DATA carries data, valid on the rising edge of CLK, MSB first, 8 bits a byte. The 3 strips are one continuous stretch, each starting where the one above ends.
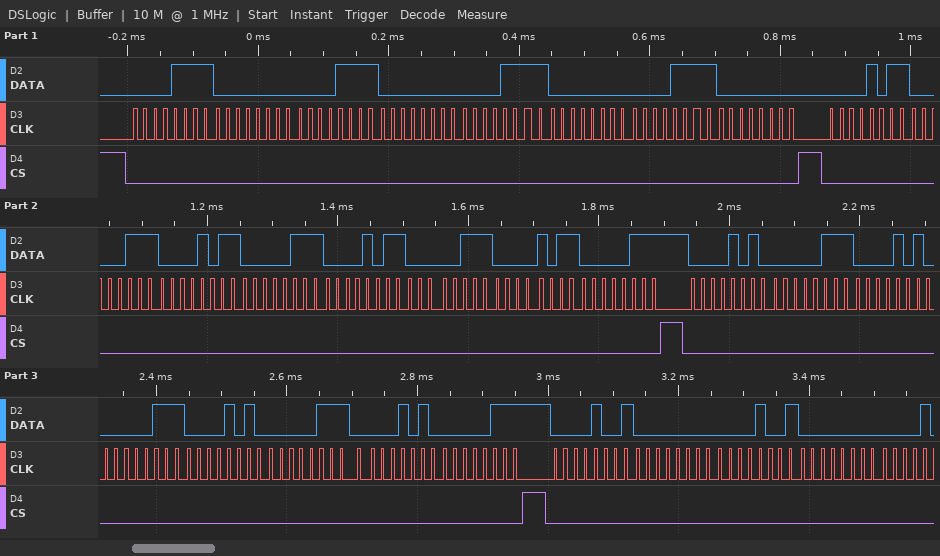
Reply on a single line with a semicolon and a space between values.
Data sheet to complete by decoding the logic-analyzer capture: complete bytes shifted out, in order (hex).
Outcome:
0x0F 0x00 0x0F 0x00 0x0F 0x00 0x0F 0x00 0x0B 0x07 0x0B 0x07 0x0B 0x07 0x0B 0x07 0x0A 0x07 0x0A 0x07 0x0A 0x07 0x0A 0x07 0x09 0x00 0x09 0x00
